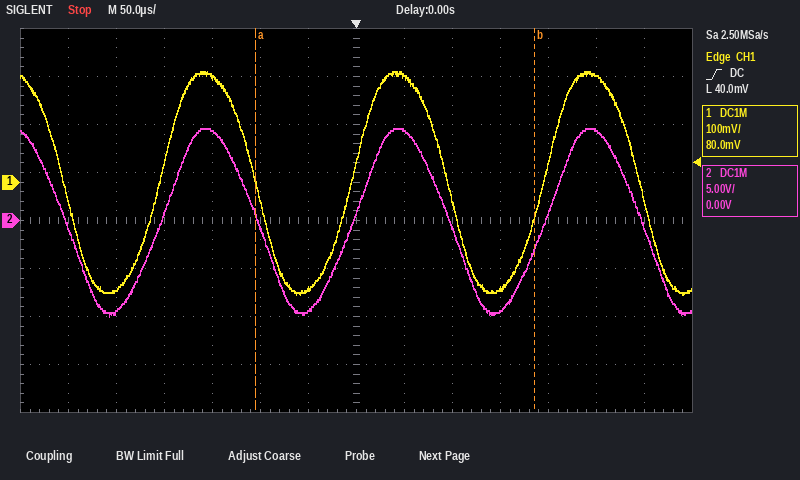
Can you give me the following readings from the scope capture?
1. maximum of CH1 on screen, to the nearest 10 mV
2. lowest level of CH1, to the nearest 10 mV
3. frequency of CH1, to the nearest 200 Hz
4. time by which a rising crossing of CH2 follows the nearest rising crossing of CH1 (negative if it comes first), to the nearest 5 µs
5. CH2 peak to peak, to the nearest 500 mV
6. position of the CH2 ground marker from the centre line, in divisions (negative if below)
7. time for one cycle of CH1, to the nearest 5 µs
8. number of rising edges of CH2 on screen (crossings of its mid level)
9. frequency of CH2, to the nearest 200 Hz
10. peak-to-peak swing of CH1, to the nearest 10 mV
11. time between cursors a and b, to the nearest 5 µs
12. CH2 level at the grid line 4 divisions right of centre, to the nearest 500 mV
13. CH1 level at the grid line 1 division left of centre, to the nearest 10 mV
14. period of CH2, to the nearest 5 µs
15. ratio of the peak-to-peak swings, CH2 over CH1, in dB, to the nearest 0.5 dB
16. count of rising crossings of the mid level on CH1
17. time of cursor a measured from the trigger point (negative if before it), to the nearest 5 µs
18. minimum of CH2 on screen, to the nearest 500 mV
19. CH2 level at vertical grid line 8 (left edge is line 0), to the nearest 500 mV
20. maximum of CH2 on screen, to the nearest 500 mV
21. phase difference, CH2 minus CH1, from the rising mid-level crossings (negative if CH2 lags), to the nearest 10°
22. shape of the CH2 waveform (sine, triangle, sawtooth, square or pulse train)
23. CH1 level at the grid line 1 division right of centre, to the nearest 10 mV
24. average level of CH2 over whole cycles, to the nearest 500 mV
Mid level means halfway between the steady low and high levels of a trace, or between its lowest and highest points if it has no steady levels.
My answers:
230 mV
-230 mV
5.0 kHz
0 µs
19.5 V
0.0 div
200 µs
3
5.0 kHz
460 mV
290 µs
500 mV
-220 mV
200 µs
32.5 dB
3
-105 µs
-10.0 V
9.5 V
9.5 V
0°
sine
220 mV
0.0 V
